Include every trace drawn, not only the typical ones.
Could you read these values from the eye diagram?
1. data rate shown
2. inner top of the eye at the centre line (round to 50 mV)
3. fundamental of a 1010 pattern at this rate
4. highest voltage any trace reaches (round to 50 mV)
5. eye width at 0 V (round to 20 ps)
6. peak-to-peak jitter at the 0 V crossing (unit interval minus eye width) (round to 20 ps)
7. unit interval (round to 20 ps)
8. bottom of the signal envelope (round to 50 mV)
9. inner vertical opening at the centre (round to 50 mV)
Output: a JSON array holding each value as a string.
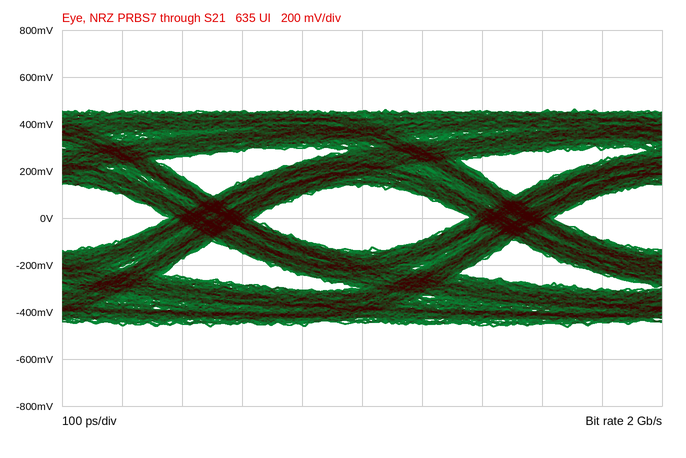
["2 Gb/s", "150 mV", "1 GHz", "450 mV", "360 ps", "140 ps", "500 ps", "-450 mV", "300 mV"]
